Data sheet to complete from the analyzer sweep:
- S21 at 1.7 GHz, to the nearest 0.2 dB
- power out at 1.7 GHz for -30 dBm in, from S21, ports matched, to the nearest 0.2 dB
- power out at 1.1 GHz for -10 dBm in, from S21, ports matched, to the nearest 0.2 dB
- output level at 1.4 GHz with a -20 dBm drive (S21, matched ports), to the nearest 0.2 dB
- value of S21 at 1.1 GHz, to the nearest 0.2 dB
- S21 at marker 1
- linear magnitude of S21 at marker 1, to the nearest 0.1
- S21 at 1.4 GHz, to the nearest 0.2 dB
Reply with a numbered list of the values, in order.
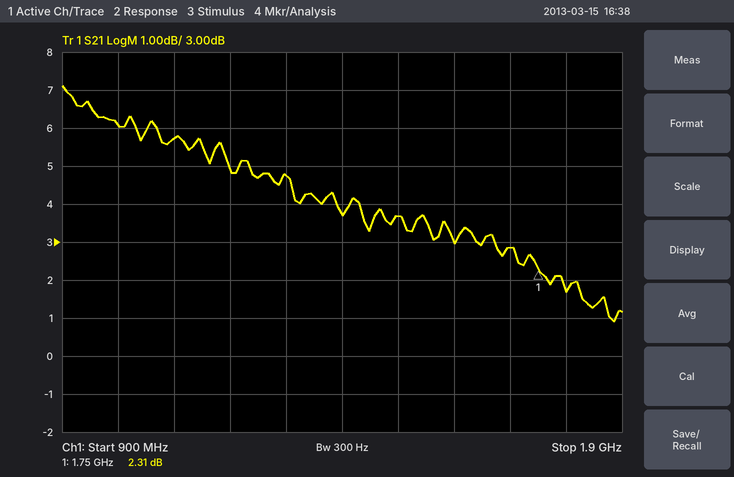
1. 2.8 dB
2. -27.2 dBm
3. -4.2 dBm
4. -16.2 dBm
5. 5.8 dB
6. 2.31 dB
7. 1.3
8. 3.8 dB
